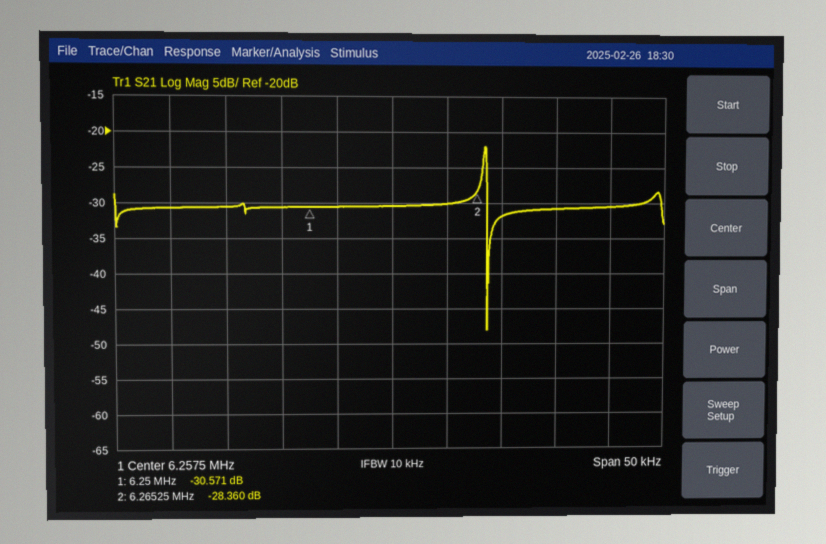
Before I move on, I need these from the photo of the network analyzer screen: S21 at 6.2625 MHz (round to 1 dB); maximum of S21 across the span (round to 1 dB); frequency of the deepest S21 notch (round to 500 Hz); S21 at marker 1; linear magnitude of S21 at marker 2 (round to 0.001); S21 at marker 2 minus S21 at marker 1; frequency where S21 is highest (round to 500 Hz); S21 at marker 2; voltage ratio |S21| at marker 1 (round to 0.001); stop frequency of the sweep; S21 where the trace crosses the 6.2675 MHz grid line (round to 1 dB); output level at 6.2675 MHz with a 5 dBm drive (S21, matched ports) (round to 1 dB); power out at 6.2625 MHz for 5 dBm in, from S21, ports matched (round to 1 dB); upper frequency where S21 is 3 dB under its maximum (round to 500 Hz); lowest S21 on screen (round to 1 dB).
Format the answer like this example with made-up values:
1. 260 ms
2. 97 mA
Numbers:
1. -30 dB
2. -22 dB
3. 6.2660 MHz
4. -30.571 dB
5. 0.038
6. 2.211 dB
7. 6.2660 MHz
8. -28.360 dB
9. 0.030
10. 6.2825 MHz
11. -32 dB
12. -27 dBm
13. -25 dBm
14. 6.2660 MHz
15. -48 dB
